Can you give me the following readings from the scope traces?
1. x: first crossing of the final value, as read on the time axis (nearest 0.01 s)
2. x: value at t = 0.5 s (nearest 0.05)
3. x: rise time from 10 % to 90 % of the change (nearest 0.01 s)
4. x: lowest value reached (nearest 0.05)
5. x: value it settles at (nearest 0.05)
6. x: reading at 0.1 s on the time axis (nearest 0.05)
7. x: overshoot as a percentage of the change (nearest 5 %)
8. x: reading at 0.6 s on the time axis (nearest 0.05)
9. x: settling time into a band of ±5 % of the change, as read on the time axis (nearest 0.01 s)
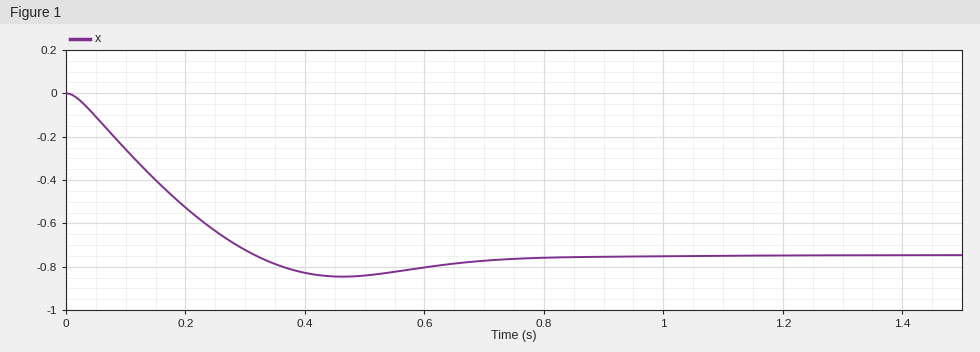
0.32 s
-0.85
0.23 s
-0.85
-0.75
-0.25
15 %
-0.80
0.66 s
